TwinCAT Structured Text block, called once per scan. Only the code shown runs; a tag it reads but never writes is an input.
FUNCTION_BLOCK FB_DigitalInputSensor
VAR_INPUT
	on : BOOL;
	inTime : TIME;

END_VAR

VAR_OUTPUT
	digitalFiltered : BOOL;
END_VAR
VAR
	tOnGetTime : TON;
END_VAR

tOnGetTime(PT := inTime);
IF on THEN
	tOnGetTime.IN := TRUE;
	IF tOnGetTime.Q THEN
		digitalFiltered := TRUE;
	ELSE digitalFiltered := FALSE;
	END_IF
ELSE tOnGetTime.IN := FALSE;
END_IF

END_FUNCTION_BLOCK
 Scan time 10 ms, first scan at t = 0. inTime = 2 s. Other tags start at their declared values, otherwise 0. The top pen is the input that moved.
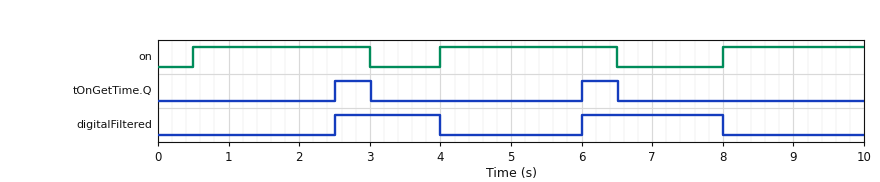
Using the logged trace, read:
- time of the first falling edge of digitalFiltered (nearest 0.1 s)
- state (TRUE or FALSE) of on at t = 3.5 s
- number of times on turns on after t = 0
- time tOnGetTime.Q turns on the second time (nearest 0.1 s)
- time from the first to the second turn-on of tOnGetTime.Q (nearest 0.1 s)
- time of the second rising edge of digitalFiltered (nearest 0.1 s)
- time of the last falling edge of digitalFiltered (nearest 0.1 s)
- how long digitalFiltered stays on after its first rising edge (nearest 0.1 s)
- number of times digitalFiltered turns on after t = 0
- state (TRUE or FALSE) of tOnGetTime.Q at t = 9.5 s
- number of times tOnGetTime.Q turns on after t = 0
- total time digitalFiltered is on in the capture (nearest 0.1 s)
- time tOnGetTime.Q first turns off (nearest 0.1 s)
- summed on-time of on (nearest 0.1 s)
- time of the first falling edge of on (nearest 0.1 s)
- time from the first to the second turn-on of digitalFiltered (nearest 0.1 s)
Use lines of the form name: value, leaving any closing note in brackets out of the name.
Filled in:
time of the first falling edge of digitalFiltered: 4.0 s
state (TRUE or FALSE) of on at t = 3.5 s: FALSE
number of times on turns on after t = 0: 3
time tOnGetTime.Q turns on the second time: 6.0 s
time from the first to the second turn-on of tOnGetTime.Q: 3.5 s
time of the second rising edge of digitalFiltered: 6.0 s
time of the last falling edge of digitalFiltered: 8.0 s
how long digitalFiltered stays on after its first rising edge: 1.5 s
number of times digitalFiltered turns on after t = 0: 2
state (TRUE or FALSE) of tOnGetTime.Q at t = 9.5 s: FALSE
number of times tOnGetTime.Q turns on after t = 0: 2
total time digitalFiltered is on in the capture: 3.5 s
time tOnGetTime.Q first turns off: 3.0 s
summed on-time of on: 7.0 s
time of the first falling edge of on: 3.0 s
time from the first to the second turn-on of digitalFiltered: 3.5 s
